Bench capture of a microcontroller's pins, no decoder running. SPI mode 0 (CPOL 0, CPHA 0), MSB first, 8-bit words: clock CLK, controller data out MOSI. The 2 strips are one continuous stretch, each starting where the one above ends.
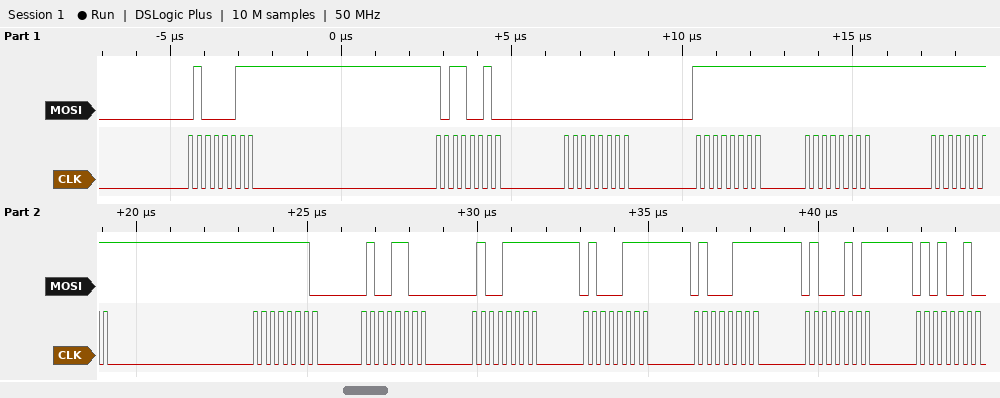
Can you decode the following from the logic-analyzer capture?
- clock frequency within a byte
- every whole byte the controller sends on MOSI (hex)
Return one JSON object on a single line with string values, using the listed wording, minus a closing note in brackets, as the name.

{"clock frequency within a byte": "4 MHz", "every whole byte the controller sends on MOSI": "0x43 0xB2 0x00 0xFF 0xFF 0xFF 0xFE 0x4C 0x4F 0x47 0x47 0x45 0x52"}
